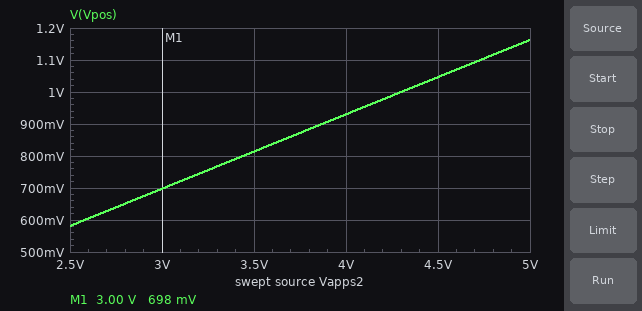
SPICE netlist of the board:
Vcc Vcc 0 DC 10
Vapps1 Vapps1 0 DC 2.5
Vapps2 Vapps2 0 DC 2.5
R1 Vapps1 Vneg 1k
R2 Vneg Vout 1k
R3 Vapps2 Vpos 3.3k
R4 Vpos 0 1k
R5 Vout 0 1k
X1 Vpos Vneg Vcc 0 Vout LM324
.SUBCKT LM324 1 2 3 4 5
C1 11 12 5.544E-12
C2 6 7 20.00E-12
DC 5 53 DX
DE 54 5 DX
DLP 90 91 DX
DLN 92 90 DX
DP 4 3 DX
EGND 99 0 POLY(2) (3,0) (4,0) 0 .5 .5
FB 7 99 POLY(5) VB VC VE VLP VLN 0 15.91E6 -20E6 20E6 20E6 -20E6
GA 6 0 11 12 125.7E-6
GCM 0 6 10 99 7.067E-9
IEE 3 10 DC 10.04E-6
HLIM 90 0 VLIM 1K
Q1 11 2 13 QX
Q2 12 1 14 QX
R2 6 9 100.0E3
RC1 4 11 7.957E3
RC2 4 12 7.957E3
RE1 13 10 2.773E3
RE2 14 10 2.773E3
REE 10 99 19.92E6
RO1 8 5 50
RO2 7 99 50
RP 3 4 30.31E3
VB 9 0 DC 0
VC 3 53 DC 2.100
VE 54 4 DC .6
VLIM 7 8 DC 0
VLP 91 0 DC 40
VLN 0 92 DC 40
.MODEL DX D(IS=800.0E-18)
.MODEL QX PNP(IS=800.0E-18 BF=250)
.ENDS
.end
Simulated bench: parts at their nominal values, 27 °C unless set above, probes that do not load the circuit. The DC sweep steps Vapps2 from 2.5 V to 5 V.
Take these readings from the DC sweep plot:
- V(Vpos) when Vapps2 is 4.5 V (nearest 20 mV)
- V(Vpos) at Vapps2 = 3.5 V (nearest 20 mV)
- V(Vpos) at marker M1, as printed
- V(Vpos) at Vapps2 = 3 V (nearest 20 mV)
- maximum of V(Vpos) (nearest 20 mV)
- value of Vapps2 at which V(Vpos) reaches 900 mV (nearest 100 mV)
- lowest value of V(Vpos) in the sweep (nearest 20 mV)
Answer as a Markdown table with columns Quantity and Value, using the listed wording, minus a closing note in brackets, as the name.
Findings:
| Quantity | Value |
|---|---|
| V(Vpos) when Vapps2 is 4.5 V | 1.04 V |
| V(Vpos) at Vapps2 = 3.5 V | 820 mV |
| V(Vpos) at marker M1, as printed | 698 mV |
| V(Vpos) at Vapps2 = 3 V | 700 mV |
| maximum of V(Vpos) | 1.16 V |
| value of Vapps2 at which V(Vpos) reaches 900 mV | 3.9 V |
| lowest value of V(Vpos) in the sweep | 580 mV |
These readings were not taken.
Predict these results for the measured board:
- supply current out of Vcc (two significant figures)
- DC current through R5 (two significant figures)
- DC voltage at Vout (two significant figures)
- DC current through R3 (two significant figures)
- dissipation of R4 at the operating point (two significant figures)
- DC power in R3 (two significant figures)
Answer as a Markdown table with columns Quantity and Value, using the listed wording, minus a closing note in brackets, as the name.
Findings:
| Quantity | Value |
|---|---|
| supply current out of Vcc | 340 µA |
| DC current through R5 | 4.2 µA |
| DC voltage at Vout | 4.2 mV |
| DC current through R3 | 580 µA |
| dissipation of R4 at the operating point | 340 µW |
| DC power in R3 | 1.1 mW |
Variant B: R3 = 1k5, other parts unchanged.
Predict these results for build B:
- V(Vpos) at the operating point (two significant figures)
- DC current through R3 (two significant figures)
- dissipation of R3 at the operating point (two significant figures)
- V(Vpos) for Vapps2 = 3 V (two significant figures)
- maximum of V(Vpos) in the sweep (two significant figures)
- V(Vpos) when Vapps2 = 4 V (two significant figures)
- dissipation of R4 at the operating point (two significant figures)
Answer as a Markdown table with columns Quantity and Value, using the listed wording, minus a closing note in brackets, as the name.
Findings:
| Quantity | Value |
|---|---|
| V(Vpos) at the operating point | 1.0 V |
| DC current through R3 | 1.0 mA |
| dissipation of R3 at the operating point | 1.5 mW |
| V(Vpos) for Vapps2 = 3 V | 1.2 V |
| maximum of V(Vpos) in the sweep | 2.0 V |
| V(Vpos) when Vapps2 = 4 V | 1.6 V |
| dissipation of R4 at the operating point | 1.0 mW |
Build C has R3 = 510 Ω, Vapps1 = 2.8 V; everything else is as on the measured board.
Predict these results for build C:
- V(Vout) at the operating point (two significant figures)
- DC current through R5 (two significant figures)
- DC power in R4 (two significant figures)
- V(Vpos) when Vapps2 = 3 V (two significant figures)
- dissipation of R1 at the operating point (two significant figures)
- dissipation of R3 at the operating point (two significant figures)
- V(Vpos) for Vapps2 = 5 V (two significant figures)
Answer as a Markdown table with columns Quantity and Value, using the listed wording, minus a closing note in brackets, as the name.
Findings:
| Quantity | Value |
|---|---|
| V(Vout) at the operating point | 510 mV |
| DC current through R5 | 510 µA |
| DC power in R4 | 2.7 mW |
| V(Vpos) when Vapps2 = 3 V | 2.0 V |
| dissipation of R1 at the operating point | 1.3 mW |
| dissipation of R3 at the operating point | 1.4 mW |
| V(Vpos) for Vapps2 = 5 V | 3.3 V |
